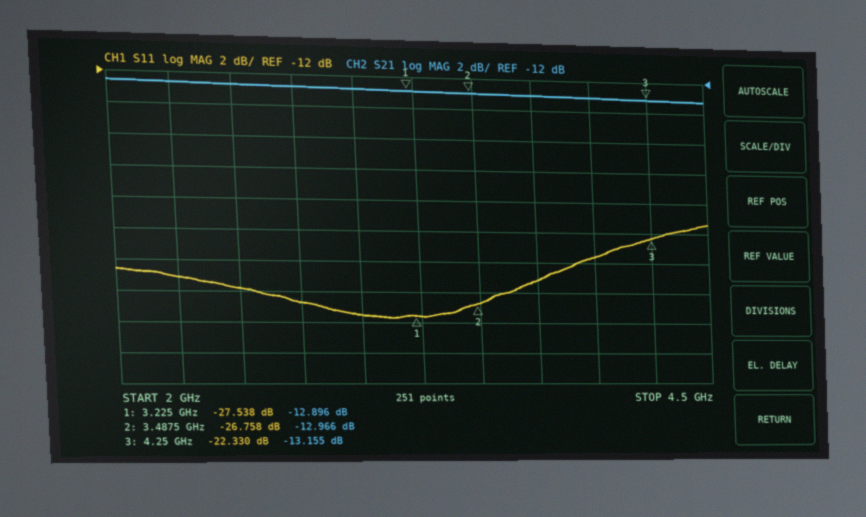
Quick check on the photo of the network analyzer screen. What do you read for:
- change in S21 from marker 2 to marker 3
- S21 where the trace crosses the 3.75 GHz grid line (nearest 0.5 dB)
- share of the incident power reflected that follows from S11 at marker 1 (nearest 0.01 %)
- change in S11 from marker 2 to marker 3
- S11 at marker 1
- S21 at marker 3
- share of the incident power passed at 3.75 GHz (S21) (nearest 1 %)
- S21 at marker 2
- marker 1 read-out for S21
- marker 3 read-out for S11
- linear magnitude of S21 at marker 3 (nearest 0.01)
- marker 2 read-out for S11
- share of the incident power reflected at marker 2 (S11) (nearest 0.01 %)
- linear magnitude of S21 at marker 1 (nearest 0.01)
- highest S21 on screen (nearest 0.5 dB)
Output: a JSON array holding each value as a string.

["-0.189 dB", "-13.0 dB", "0.18 %", "4.428 dB", "-27.538 dB", "-13.155 dB", "5 %", "-12.966 dB", "-12.896 dB", "-22.330 dB", "0.22", "-26.758 dB", "0.21 %", "0.23", "-12.5 dB"]
